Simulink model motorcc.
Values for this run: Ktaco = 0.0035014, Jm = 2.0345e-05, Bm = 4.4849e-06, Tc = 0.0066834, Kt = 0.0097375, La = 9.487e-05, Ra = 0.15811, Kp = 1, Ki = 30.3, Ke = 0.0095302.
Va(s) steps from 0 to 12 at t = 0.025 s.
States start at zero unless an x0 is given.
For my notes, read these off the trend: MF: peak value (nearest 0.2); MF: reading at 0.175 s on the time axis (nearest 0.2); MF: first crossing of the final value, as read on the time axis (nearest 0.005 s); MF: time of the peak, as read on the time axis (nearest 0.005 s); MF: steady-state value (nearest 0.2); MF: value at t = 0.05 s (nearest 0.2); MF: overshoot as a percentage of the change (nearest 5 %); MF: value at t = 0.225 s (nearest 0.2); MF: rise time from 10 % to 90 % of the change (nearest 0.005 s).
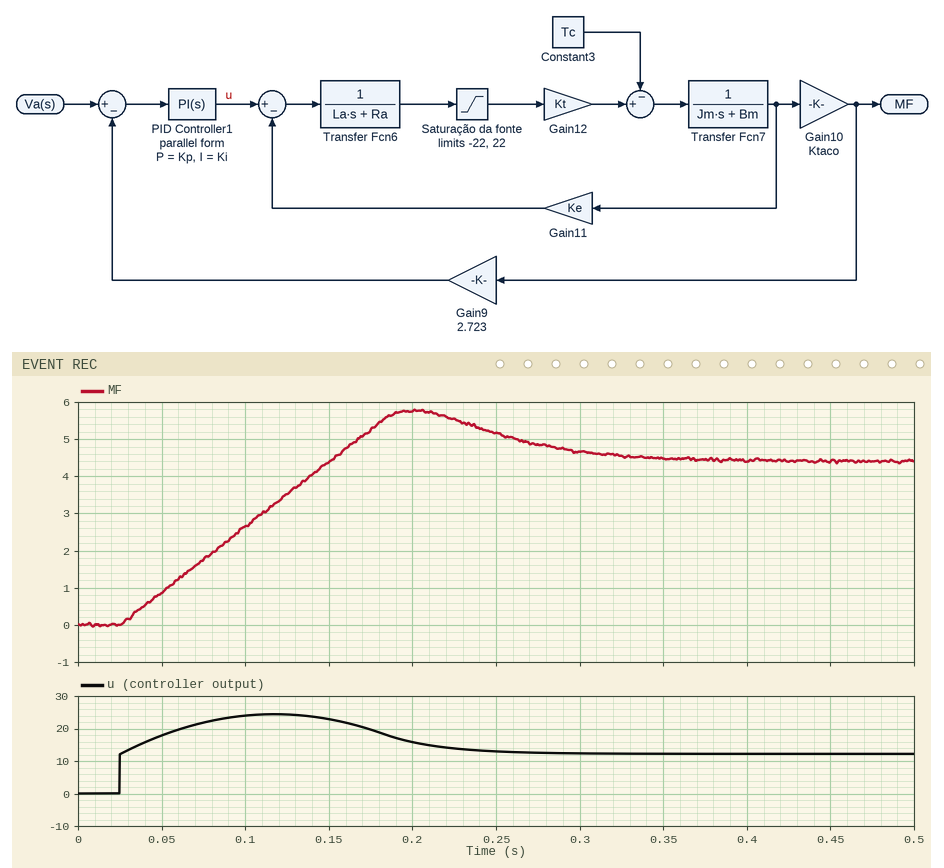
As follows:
5.8
5.2
0.150 s
0.200 s
4.4
0.8
30 %
5.6
0.100 s
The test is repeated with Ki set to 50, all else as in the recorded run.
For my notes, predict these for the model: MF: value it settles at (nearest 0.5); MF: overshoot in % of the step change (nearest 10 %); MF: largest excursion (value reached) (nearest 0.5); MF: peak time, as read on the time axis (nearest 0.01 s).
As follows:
4.5
50 %
7.0
0.22 s
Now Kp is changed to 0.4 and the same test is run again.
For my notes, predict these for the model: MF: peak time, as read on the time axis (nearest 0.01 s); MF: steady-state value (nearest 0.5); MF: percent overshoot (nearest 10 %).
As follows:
0.21 s
4.5
40 %
